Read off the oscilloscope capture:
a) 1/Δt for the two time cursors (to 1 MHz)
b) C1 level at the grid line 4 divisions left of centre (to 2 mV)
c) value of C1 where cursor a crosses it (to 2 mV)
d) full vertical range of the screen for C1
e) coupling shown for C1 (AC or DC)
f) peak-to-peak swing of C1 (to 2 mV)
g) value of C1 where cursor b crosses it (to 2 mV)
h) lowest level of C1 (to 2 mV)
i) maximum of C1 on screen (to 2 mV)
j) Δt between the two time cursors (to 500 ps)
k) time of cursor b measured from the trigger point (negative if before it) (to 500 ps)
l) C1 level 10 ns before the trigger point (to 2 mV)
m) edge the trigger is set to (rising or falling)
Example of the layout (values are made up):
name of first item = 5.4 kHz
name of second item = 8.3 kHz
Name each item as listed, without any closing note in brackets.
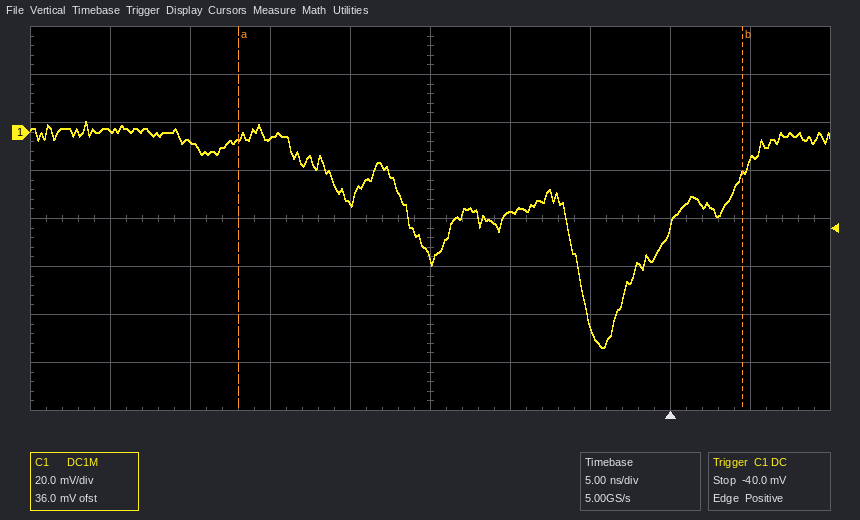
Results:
1/Δt for the two time cursors = 32 MHz
C1 level at the grid line 4 divisions left of centre = 0 mV
value of C1 where cursor a crosses it = -2 mV
full vertical range of the screen for C1 = 160 mV
coupling shown for C1 = DC
peak-to-peak swing of C1 = 94 mV
value of C1 where cursor b crosses it = -18 mV
lowest level of C1 = -90 mV
maximum of C1 on screen = 4 mV
Δt between the two time cursors = 31.5 ns
time of cursor b measured from the trigger point (negative if before it) = +4.5 ns
C1 level 10 ns before the trigger point = -34 mV
edge the trigger is set to = rising
